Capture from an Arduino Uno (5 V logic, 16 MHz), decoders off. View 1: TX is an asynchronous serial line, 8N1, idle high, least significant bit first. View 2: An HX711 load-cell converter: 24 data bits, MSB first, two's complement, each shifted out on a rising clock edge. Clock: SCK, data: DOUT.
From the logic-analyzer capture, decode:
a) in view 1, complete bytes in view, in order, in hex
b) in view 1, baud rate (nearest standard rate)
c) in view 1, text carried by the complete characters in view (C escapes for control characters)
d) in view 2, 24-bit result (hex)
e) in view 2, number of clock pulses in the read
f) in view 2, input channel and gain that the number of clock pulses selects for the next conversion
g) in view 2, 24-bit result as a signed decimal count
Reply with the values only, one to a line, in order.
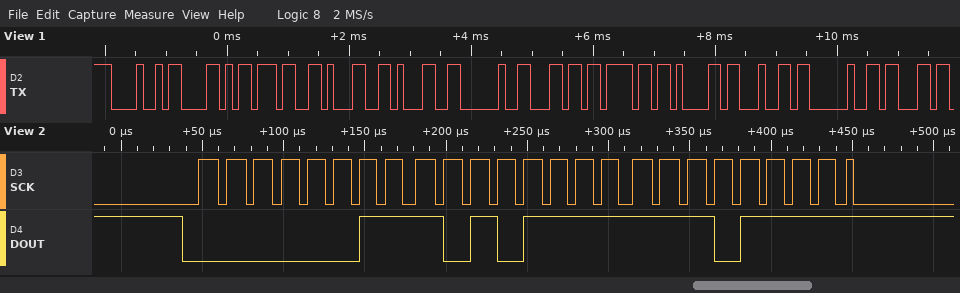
48 58 37 31 31 20 6C 6F 61 64 20 63
9600 baud
"HX711 load c"
0x03AFEF
25
channel A, gain 128
241647
